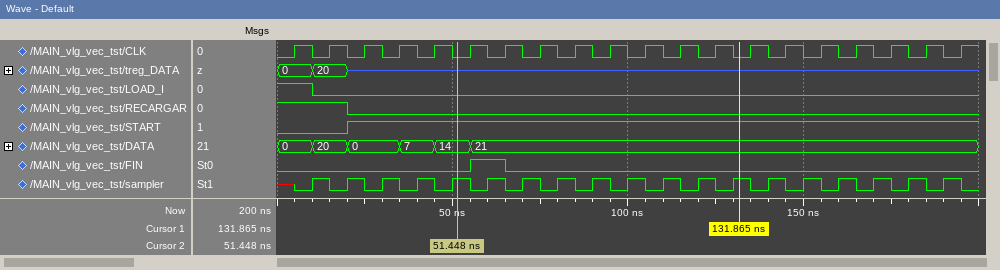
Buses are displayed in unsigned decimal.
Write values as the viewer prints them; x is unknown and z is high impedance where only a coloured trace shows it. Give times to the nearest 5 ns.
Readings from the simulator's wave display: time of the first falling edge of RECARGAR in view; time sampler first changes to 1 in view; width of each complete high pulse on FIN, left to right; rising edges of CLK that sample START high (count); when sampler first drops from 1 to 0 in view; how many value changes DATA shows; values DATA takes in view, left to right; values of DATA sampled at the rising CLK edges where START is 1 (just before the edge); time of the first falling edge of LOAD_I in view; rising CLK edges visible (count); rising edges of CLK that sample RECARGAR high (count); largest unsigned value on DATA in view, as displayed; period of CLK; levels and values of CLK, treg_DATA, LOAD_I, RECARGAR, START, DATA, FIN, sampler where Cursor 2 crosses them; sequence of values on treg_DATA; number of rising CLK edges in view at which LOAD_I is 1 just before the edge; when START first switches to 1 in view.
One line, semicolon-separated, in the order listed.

20 ns; 10 ns; 10 ns; 18; 15 ns; 5; 0, 20, 0, 7, 14, 21; 0, 0, 7, 14, 21, 21, 21, 21, 21, 21, 21, 21, 21, 21, 21, 21, 21, 21; 10 ns; 20; 2; 21; 10 ns; CLK=0, treg_DATA=z, LOAD_I=0, RECARGAR=0, START=1, DATA=14, FIN=0, sampler=1; 0, 20, z; 1; 20 ns
